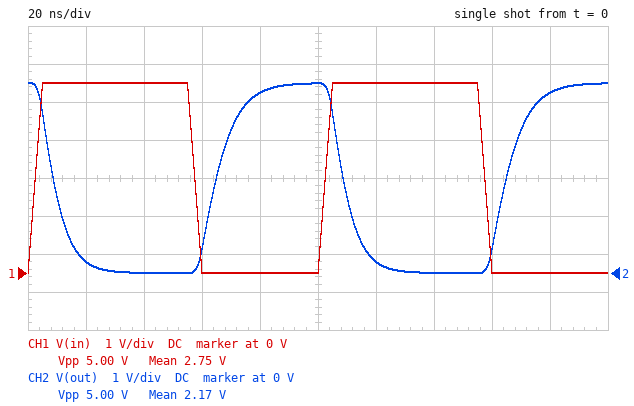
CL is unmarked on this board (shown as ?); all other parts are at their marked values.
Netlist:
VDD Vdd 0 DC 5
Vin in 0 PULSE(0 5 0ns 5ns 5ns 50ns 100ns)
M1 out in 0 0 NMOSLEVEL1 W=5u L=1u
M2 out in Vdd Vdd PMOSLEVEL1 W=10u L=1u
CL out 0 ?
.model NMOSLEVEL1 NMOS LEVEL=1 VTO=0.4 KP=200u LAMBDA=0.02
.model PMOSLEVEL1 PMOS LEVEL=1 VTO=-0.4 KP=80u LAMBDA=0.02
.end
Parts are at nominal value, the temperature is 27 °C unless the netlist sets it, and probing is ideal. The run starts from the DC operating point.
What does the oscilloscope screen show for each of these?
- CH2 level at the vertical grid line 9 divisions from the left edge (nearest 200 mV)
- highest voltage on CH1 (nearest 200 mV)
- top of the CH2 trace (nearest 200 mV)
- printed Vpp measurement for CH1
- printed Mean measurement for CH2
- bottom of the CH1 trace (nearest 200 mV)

4.8 V
5.0 V
5.0 V
5.00 V
2.17 V
0 V
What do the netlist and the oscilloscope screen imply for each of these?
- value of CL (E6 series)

22 pF
